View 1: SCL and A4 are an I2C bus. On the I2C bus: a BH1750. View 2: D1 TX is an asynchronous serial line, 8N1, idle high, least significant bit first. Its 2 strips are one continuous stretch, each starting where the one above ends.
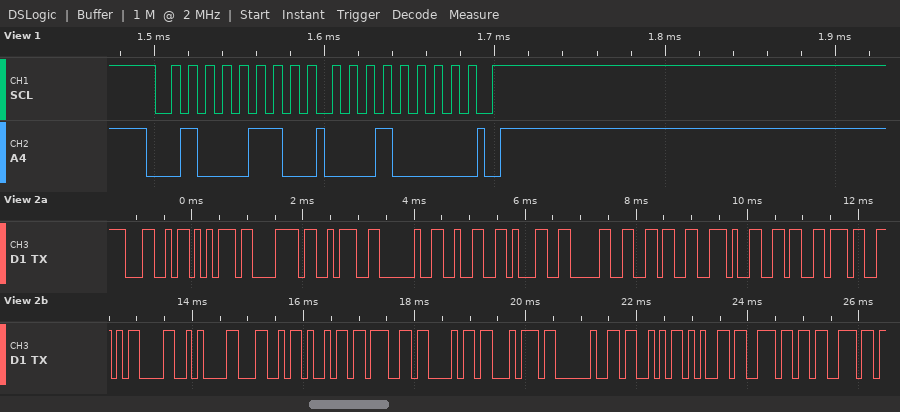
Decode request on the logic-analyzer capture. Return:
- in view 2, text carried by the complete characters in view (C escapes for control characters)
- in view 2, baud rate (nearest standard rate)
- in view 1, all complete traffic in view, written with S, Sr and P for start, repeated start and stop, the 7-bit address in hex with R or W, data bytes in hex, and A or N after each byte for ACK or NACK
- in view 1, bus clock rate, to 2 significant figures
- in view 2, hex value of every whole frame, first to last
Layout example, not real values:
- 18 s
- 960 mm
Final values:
- "Lux: 2106.67\r\nLight Sens"
- 9600 baud
- S 23W A 10 A P
- 100 kHz
- 4C 75 78 3A 20 32 31 30 36 2E 36 37 0D 0A 4C 69 67 68 74 20 53 65 6E 73
